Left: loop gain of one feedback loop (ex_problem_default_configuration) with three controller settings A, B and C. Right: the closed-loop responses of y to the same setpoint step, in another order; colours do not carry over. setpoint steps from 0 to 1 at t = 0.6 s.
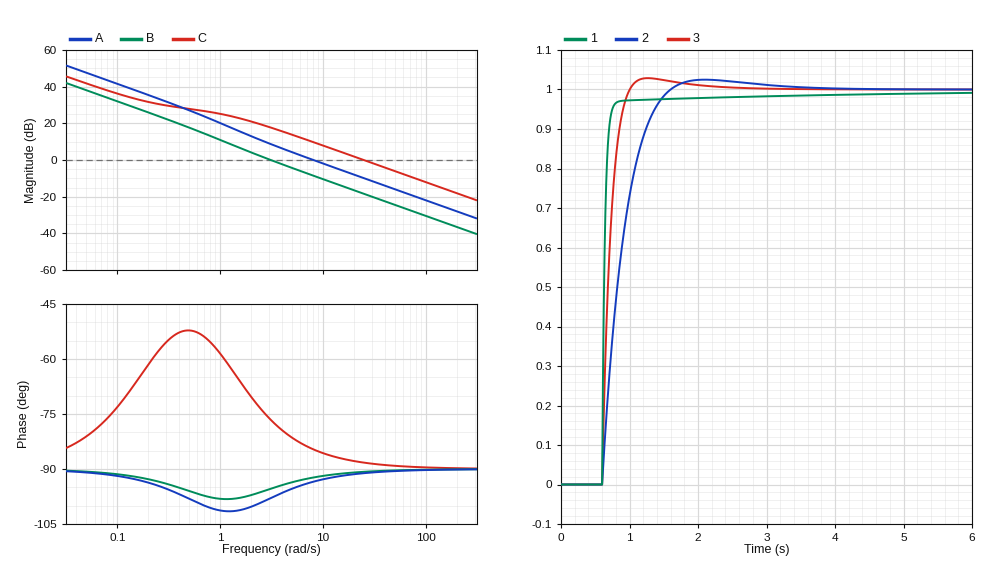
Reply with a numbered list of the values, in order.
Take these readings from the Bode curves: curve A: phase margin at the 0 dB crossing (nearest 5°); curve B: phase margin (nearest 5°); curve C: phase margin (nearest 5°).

1. 85°
2. 85°
3. 90°
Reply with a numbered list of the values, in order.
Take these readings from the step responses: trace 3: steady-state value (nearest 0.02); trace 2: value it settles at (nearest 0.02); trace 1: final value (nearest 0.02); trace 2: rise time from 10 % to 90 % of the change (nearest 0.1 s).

1. 1.00
2. 1.00
3. 1.00
4. 0.6 s
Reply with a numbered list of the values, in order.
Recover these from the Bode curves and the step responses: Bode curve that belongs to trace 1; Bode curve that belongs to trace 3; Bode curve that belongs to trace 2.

1. C
2. A
3. B
